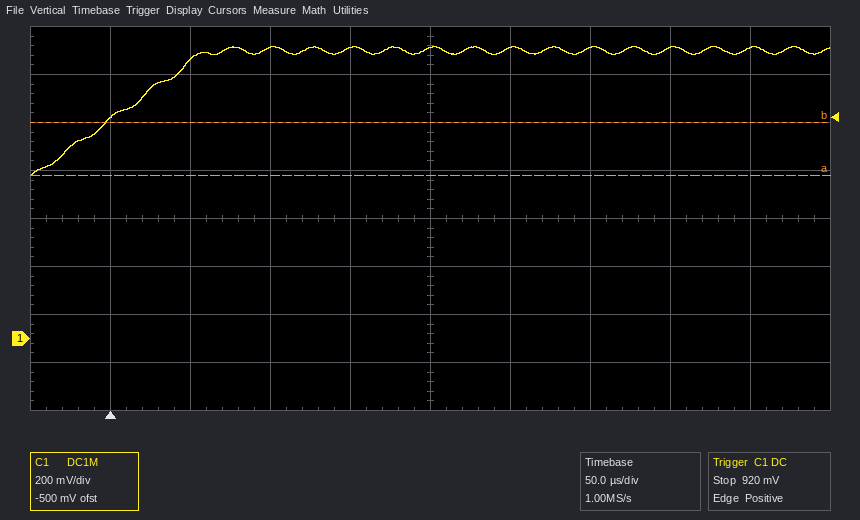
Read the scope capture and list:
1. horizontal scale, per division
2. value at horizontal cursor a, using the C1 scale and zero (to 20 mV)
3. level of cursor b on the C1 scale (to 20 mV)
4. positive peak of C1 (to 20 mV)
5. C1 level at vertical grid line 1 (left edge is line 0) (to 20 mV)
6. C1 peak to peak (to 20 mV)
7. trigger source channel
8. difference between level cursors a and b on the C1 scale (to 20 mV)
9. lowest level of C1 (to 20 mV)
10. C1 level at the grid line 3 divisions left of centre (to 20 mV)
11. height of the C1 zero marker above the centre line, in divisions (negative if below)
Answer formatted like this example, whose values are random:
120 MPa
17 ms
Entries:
50 µs
680 mV
900 mV
1.22 V
920 mV
540 mV
C1
220 mV
680 mV
1.16 V
-2.5 div
